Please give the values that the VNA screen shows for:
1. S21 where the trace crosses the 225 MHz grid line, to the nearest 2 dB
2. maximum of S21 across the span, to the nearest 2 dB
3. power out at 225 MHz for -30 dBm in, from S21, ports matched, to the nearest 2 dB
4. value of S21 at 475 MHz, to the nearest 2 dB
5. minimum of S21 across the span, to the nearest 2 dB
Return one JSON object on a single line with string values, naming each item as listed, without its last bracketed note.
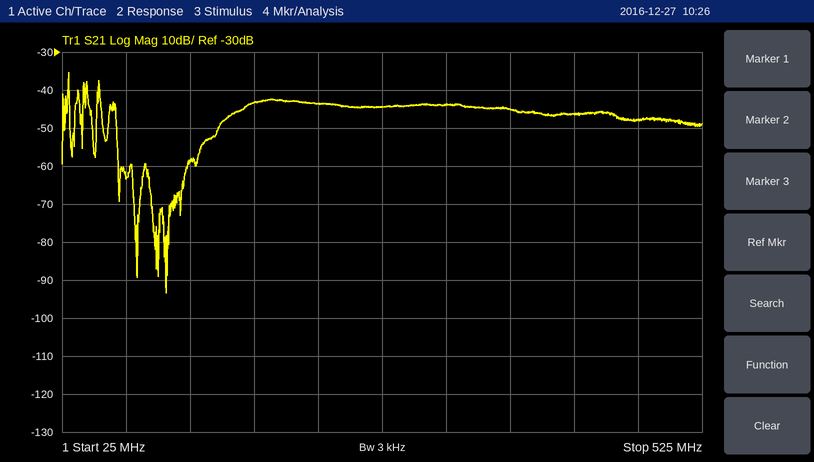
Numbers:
{"S21 where the trace crosses the 225 MHz grid line, to the nearest 2 dB": "-44 dB", "maximum of S21 across the span, to the nearest 2 dB": "-36 dB", "power out at 225 MHz for -30 dBm in, from S21, ports matched, to the nearest 2 dB": "-74 dBm", "value of S21 at 475 MHz, to the nearest 2 dB": "-48 dB", "minimum of S21 across the span, to the nearest 2 dB": "-94 dB"}
